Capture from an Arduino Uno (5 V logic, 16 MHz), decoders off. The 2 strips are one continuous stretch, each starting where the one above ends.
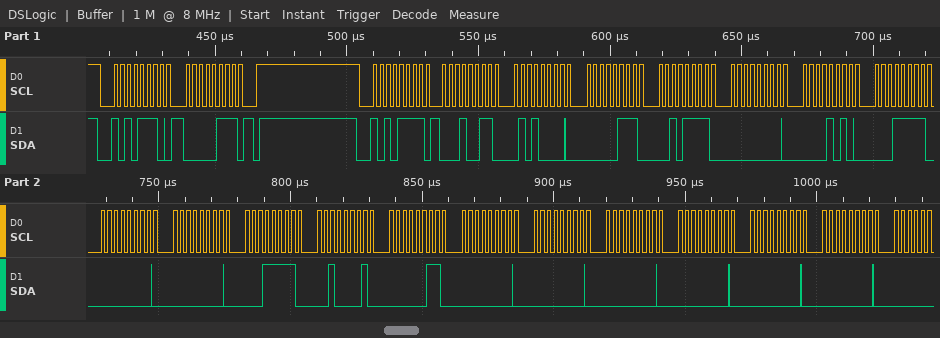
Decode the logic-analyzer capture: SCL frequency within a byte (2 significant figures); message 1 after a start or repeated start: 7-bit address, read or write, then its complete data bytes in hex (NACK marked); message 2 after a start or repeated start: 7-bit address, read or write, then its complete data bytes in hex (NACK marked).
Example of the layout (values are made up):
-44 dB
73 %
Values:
400 kHz
0x57 write: 07
0x57 read: 13 50 07 2F 00 0A 1F 00 00 1F 21 03 00 00 00 00 00 00
